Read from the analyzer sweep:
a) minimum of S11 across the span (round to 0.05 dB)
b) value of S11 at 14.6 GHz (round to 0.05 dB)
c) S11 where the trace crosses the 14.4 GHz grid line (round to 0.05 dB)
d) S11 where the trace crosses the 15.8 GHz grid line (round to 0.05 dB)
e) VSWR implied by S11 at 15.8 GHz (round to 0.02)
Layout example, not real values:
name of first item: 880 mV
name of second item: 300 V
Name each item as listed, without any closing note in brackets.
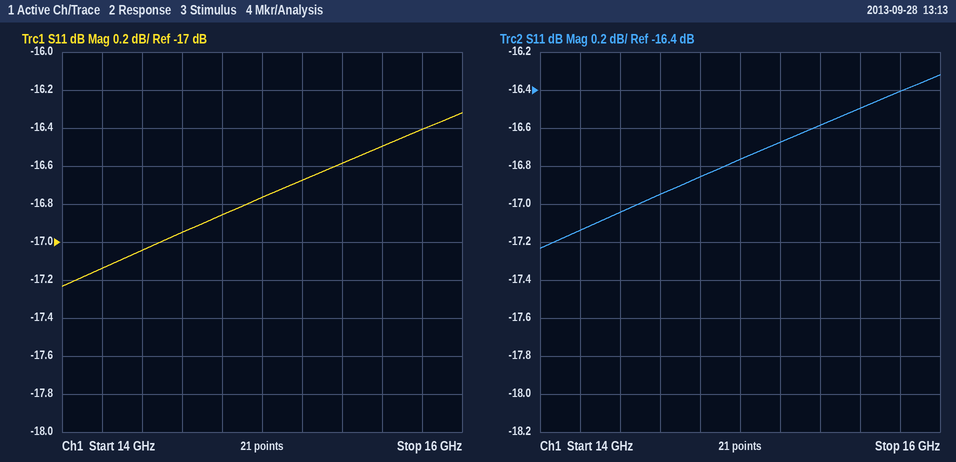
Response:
minimum of S11 across the span: -17.25 dB
value of S11 at 14.6 GHz: -16.95 dB
S11 where the trace crosses the 14.4 GHz grid line: -17.05 dB
S11 where the trace crosses the 15.8 GHz grid line: -16.40 dB
VSWR implied by S11 at 15.8 GHz: 1.36
